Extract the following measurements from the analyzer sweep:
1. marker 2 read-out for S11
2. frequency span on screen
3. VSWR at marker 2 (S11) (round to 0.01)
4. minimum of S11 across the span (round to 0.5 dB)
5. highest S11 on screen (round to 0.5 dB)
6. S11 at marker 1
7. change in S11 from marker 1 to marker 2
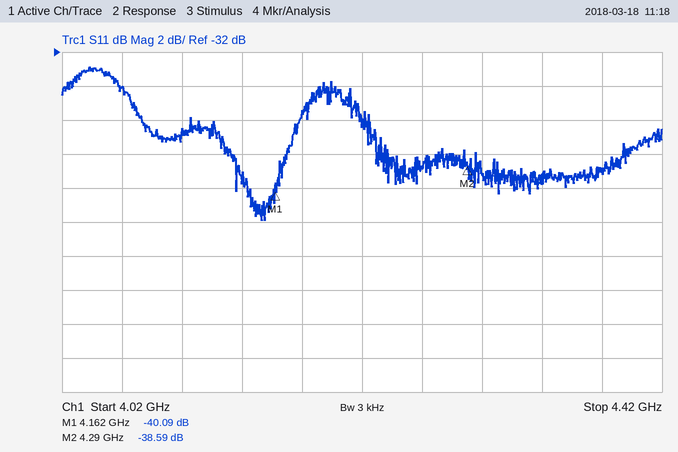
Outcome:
-38.59 dB
400 MHz
1.02
-42.0 dB
-33.0 dB
-40.09 dB
1.50 dB
